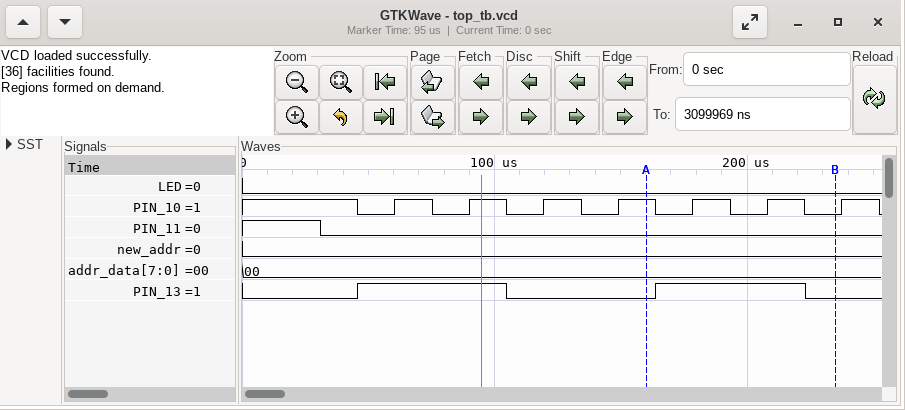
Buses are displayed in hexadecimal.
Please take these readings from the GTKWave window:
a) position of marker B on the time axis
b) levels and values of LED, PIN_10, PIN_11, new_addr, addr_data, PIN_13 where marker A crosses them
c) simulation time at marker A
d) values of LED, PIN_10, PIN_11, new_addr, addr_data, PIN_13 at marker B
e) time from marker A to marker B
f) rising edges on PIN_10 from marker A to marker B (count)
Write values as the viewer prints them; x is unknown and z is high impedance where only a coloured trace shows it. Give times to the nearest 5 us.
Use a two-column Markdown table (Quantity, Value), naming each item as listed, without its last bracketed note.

| Quantity | Value |
|---|---|
| position of marker B on the time axis | 235 us |
| levels and values of LED, PIN_10, PIN_11, new_addr, addr_data, PIN_13 where marker A crosses them | LED=0, PIN_10=1, PIN_11=0, new_addr=0, addr_data=00, PIN_13=0 |
| simulation time at marker A | 160 us |
| values of LED, PIN_10, PIN_11, new_addr, addr_data, PIN_13 at marker B | LED=0, PIN_10=0, PIN_11=0, new_addr=0, addr_data=00, PIN_13=0 |
| time from marker A to marker B | 75 us |
| rising edges on PIN_10 from marker A to marker B | 2 |
